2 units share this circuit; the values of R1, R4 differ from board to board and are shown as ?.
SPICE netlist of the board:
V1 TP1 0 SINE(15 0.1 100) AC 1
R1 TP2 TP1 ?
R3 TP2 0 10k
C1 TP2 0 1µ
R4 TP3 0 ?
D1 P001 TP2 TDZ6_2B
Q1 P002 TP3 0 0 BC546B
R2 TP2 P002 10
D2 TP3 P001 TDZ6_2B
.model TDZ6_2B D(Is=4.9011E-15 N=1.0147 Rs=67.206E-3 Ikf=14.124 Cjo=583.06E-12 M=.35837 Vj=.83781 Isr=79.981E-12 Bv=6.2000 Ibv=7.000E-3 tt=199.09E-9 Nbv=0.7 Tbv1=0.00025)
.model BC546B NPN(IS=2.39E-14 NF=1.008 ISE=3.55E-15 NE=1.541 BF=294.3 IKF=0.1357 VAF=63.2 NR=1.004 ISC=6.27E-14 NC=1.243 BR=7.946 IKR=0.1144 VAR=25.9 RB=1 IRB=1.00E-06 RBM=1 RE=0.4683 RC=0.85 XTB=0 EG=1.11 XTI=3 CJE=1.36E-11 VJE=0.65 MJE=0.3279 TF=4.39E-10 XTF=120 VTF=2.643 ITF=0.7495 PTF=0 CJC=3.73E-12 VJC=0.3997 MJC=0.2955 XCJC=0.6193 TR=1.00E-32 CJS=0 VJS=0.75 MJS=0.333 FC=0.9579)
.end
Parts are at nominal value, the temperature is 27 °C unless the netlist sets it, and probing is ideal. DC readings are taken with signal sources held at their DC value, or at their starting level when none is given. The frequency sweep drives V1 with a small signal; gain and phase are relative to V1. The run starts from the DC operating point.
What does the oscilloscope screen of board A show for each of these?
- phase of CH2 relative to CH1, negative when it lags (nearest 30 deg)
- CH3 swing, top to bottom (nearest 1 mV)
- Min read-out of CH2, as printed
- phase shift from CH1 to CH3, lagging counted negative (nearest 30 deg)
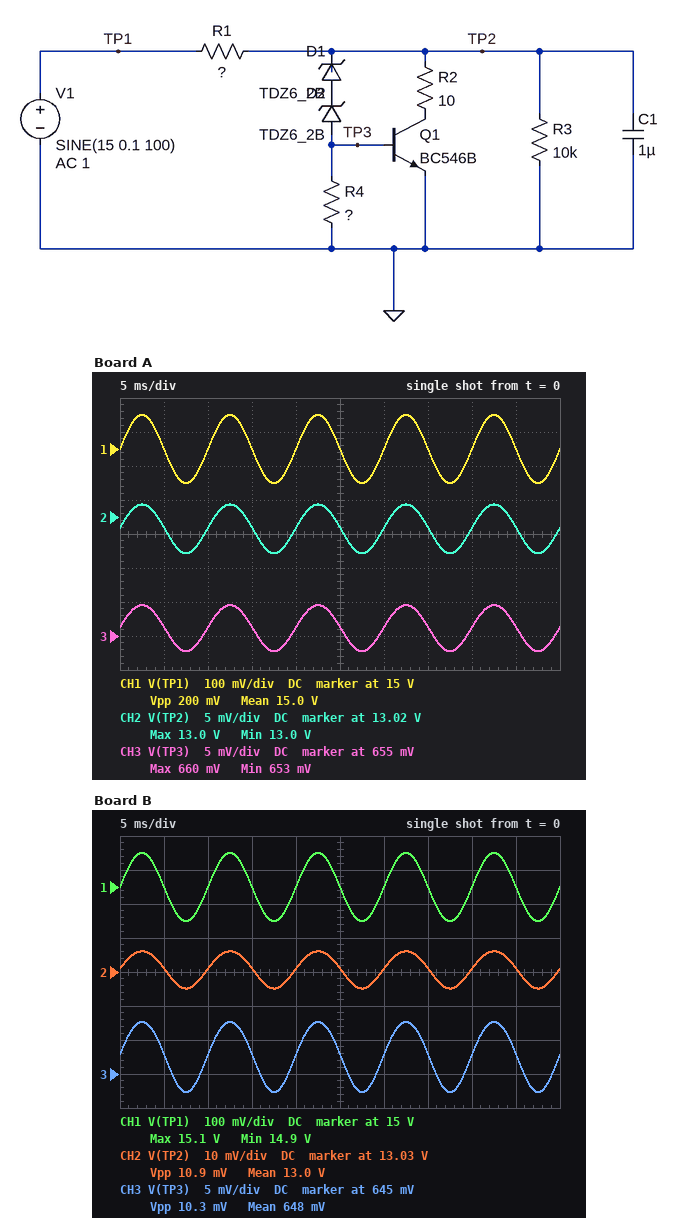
0 deg
7 mV
13.0 V
0 deg
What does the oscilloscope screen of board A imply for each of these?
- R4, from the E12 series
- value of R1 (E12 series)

270 Ω
330 Ω
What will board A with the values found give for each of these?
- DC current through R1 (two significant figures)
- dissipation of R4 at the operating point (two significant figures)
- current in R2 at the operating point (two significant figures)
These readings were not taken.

6.0 mA
1.6 mW
2.3 mA
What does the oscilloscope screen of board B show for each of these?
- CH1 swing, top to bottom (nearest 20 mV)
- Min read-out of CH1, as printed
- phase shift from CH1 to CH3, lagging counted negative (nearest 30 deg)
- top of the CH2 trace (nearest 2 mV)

200 mV
14.9 V
0 deg
13.036 V
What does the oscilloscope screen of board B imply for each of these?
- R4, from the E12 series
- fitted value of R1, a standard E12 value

150 Ω
270 Ω
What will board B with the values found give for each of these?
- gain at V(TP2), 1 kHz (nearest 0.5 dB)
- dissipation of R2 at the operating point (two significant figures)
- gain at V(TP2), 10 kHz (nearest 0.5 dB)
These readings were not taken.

-25.5 dB
28 µW
-28.0 dB
